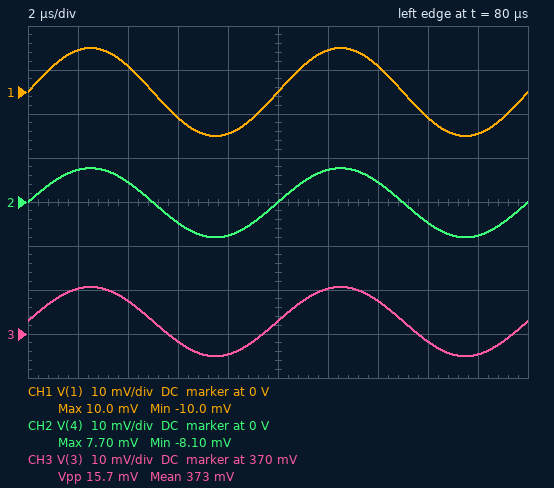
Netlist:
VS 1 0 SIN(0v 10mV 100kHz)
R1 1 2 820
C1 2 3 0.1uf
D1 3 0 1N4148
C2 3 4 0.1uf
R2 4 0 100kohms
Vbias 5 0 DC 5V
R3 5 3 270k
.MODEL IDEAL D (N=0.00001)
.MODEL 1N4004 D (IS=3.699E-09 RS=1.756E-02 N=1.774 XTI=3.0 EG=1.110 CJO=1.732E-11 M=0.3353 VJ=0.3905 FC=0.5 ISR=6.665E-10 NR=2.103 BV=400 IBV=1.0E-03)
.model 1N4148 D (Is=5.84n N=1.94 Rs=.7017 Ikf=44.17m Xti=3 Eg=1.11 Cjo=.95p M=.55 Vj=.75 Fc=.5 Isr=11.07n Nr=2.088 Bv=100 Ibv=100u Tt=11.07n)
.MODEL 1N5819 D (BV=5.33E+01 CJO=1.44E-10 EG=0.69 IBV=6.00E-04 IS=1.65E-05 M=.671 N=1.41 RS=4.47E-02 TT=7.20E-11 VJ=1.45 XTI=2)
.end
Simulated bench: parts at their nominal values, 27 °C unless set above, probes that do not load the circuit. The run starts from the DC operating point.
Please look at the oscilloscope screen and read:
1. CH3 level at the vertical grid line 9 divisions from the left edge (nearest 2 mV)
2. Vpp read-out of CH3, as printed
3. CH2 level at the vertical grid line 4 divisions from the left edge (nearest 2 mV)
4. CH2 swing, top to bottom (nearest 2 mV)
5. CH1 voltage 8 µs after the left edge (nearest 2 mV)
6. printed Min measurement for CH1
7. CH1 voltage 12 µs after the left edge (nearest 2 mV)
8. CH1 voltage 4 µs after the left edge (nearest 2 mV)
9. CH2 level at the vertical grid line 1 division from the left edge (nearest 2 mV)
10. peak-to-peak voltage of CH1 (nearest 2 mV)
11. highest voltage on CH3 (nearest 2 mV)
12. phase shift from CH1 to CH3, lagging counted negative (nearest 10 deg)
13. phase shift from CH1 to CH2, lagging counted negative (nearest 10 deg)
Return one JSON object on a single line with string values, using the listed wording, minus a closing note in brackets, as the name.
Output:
{"CH3 level at the vertical grid line 9 divisions from the left edge": "366 mV", "Vpp read-out of CH3, as printed": "15.7 mV", "CH2 level at the vertical grid line 4 divisions from the left edge": "-8 mV", "CH2 swing, top to bottom": "16 mV", "CH1 voltage 8 µs after the left edge": "-10 mV", "printed Min measurement for CH1": "-10.0 mV", "CH1 voltage 12 µs after the left edge": "10 mV", "CH1 voltage 4 µs after the left edge": "6 mV", "CH2 level at the vertical grid line 1 division from the left edge": "8 mV", "peak-to-peak voltage of CH1": "20 mV", "highest voltage on CH3": "380 mV", "phase shift from CH1 to CH3, lagging counted negative": "0 deg", "phase shift from CH1 to CH2, lagging counted negative": "0 deg"}
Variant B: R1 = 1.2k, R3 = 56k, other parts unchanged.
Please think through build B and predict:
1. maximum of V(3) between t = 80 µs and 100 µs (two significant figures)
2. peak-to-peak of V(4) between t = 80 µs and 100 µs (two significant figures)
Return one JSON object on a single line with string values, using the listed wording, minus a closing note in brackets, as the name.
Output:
{"maximum of V(3) between t = 80 µs and 100 µs": "460 mV", "peak-to-peak of V(4) between t = 80 µs and 100 µs": "7.1 mV"}
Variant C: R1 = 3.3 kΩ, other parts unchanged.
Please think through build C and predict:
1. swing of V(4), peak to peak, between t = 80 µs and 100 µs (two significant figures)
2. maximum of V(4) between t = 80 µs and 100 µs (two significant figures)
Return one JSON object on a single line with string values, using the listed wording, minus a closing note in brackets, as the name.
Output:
{"swing of V(4), peak to peak, between t = 80 µs and 100 µs": "9.6 mV", "maximum of V(4) between t = 80 µs and 100 µs": "4.7 mV"}
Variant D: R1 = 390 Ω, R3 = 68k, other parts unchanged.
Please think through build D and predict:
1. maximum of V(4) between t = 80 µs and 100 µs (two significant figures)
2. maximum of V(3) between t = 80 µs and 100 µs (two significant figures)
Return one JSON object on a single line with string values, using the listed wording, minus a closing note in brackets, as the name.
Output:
{"maximum of V(4) between t = 80 µs and 100 µs": "6.5 mV", "maximum of V(3) between t = 80 µs and 100 µs": "450 mV"}
